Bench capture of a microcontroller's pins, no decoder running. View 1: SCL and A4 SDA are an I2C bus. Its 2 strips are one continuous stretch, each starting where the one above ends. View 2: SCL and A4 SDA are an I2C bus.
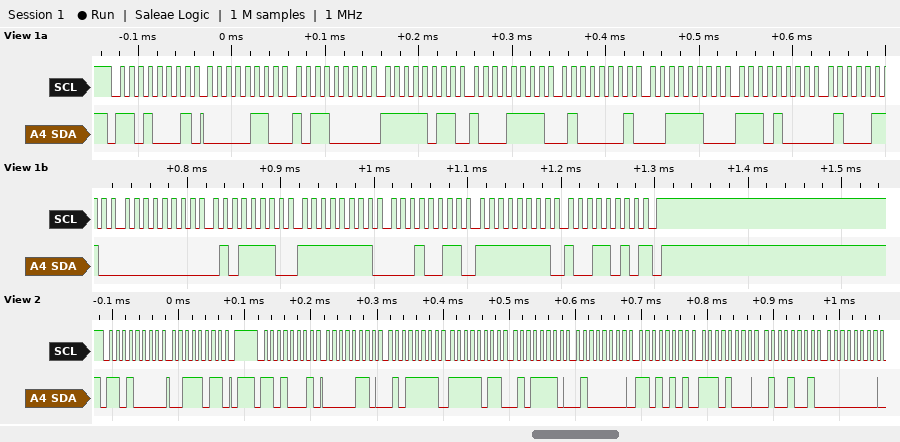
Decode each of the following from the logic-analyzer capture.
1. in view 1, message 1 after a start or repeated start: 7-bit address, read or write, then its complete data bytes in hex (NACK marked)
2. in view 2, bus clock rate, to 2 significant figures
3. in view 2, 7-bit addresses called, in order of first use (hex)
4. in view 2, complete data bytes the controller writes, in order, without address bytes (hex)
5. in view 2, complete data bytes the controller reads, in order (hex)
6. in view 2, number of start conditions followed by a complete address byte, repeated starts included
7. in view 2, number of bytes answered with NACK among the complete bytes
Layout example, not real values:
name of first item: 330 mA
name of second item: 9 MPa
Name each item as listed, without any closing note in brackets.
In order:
in view 1, message 1 after a start or repeated start: 7-bit address, read or write, then its complete data bytes in hex: 0x68 read: 06 B0 FB 8F 41 3C E8 46 00 5E FF 13 FF 9A NACK
in view 2, bus clock rate, to 2 significant figures: 100 kHz
in view 2, 7-bit addresses called, in order of first use: 0x68
in view 2, complete data bytes the controller writes, in order, without address bytes: 3B
in view 2, complete data bytes the controller reads, in order: 06 5F FB 5E 40 D5 E8 49 00
in view 2, number of start conditions followed by a complete address byte, repeated starts included: 2
in view 2, number of bytes answered with NACK among the complete bytes: 0
